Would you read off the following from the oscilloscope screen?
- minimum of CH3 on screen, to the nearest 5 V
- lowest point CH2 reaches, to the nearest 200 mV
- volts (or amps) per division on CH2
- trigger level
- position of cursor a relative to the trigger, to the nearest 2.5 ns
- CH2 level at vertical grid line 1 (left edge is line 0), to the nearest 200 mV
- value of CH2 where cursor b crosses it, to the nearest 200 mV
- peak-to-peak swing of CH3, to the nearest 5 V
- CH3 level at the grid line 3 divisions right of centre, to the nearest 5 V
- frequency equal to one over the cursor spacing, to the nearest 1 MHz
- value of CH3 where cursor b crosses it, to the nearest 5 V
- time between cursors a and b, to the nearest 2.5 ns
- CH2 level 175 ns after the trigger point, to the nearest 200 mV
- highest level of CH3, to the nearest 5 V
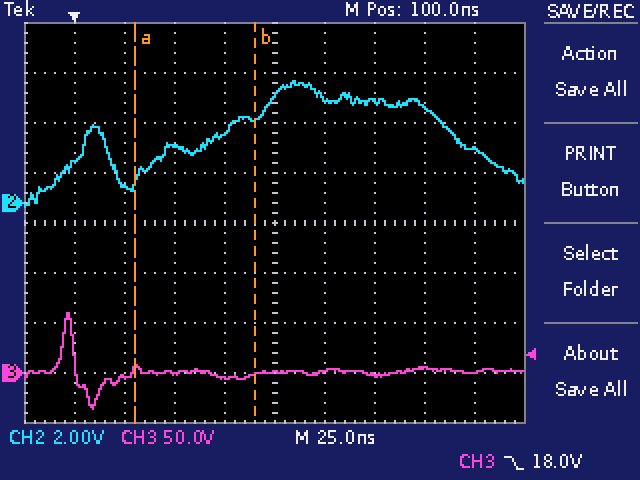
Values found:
-35 V
-200 mV
2 V
18.0 V
+30.0 ns
1.6 V
3.4 V
95 V
5 V
17 MHz
0 V
60.0 ns
3.8 V
60 V
